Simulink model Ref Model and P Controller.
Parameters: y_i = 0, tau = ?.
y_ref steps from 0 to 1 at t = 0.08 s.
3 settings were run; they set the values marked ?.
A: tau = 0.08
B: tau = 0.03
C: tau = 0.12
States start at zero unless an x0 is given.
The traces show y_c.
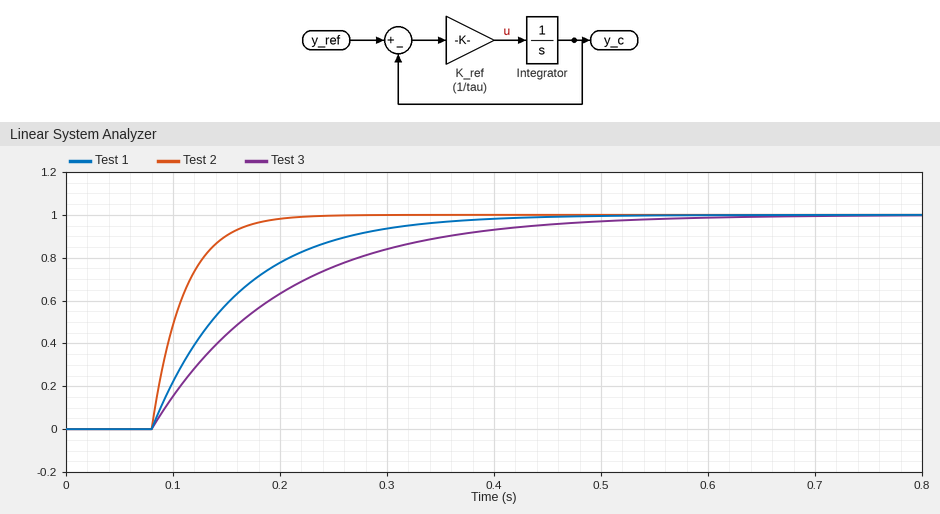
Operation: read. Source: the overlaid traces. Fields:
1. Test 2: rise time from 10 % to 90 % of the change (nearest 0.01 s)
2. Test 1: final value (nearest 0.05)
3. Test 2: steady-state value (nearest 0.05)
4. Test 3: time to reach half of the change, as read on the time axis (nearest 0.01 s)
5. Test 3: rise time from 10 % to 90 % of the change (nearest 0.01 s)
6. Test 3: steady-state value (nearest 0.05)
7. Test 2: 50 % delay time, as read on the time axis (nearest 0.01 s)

0.07 s
1.00
1.00
0.16 s
0.26 s
1.00
0.10 s
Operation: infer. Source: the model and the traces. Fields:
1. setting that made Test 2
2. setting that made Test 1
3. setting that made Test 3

B
A
C
